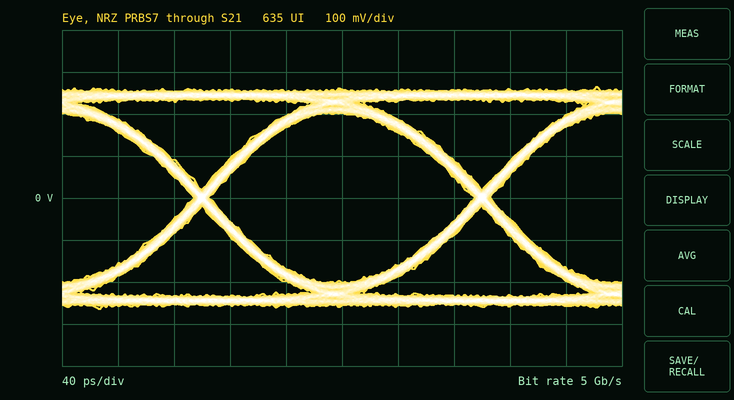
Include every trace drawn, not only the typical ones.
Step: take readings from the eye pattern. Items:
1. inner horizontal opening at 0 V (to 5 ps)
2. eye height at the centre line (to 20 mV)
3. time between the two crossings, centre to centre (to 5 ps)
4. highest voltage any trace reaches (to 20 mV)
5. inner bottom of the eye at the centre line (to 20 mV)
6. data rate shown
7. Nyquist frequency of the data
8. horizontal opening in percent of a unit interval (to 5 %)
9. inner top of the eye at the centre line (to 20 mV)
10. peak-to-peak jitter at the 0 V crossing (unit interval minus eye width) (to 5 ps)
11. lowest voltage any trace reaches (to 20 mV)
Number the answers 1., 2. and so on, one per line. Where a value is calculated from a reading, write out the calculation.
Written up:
1. 190 ps
2. 400 mV
3. 200 ps
4. 260 mV
5. -200 mV
6. 5 Gb/s
7. 2.5 GHz
8. 190 ps / 200 ps ≈ 95 %
9. 200 mV
10. 10 ps
11. -260 mV
